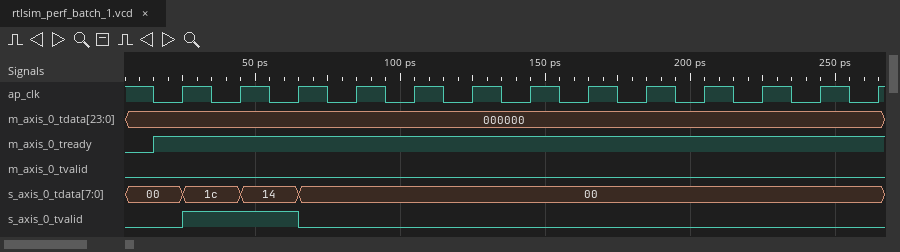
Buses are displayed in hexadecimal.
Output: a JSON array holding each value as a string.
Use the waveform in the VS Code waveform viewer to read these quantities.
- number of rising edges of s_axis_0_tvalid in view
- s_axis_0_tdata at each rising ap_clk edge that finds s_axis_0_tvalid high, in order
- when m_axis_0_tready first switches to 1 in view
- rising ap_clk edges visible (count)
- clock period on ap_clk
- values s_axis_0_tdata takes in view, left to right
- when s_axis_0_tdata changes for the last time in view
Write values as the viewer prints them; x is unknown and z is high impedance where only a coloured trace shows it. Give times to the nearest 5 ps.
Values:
["1", "1c, 14", "15 ps", "13", "20 ps", "00, 1c, 14, 00", "65 ps"]
